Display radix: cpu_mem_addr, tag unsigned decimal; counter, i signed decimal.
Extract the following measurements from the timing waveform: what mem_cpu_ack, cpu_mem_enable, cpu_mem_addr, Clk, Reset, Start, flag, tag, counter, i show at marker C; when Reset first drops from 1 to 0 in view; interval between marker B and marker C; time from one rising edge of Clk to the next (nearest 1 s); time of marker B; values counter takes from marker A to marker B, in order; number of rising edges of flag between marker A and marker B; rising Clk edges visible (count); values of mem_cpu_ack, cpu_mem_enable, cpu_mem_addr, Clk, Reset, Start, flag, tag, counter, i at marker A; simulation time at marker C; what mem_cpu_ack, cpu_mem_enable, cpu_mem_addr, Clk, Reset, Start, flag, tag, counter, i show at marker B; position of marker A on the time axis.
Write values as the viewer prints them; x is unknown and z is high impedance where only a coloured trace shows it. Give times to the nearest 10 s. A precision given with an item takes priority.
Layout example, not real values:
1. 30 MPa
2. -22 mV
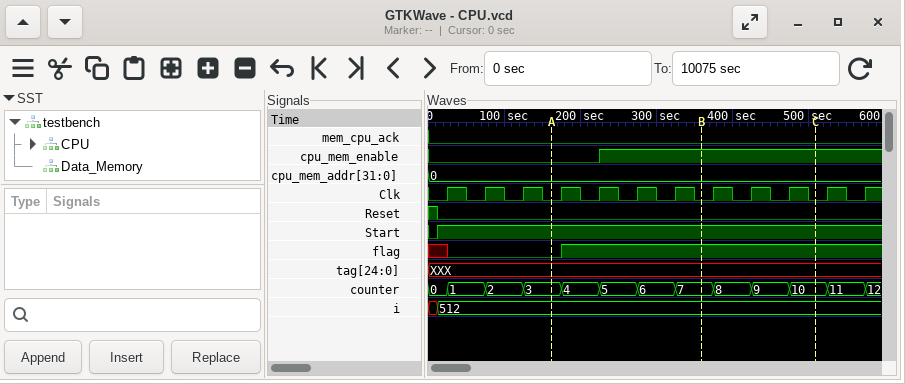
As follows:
1. mem_cpu_ack=0, cpu_mem_enable=1, cpu_mem_addr=0, Clk=0, Reset=0, Start=1, flag=1, tag=XXX, counter=10, i=512
2. 10 s
3. 150 s
4. 50 s
5. 360 s
6. 3, 4, 5, 6, 7
7. 1
8. 12
9. mem_cpu_ack=0, cpu_mem_enable=0, cpu_mem_addr=0, Clk=0, Reset=0, Start=1, flag=0, tag=XXX, counter=3, i=512
10. 510 s
11. mem_cpu_ack=0, cpu_mem_enable=1, cpu_mem_addr=0, Clk=0, Reset=0, Start=1, flag=1, tag=XXX, counter=7, i=512
12. 160 s
